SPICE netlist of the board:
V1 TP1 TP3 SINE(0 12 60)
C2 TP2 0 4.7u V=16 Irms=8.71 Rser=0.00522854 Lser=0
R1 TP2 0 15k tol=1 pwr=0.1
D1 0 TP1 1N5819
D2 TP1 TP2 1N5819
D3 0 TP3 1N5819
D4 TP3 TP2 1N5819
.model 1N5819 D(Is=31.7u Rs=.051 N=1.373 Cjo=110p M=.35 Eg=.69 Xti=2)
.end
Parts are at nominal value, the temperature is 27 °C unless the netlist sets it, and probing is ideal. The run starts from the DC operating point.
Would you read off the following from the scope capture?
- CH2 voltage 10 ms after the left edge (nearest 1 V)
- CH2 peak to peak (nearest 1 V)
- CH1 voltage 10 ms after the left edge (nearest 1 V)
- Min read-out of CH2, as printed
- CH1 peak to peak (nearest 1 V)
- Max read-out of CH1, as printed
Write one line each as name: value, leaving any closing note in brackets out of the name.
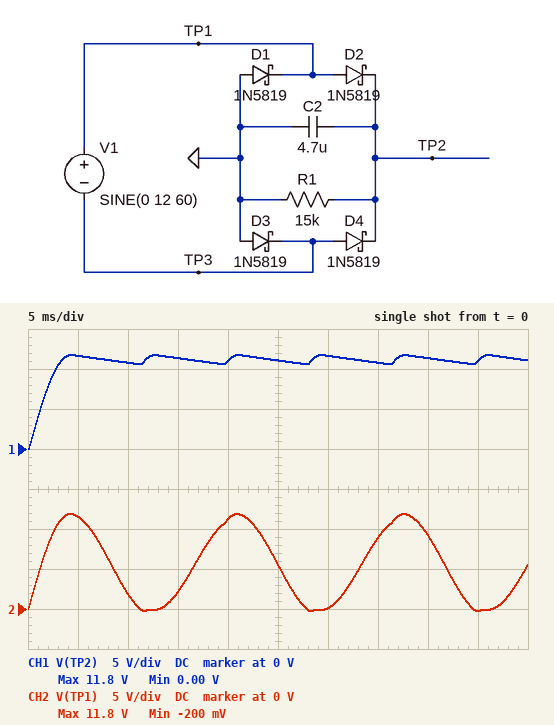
CH2 voltage 10 ms after the left edge: 2 V
CH2 peak to peak: 12 V
CH1 voltage 10 ms after the left edge: 11 V
Min read-out of CH2, as printed: -200 mV
CH1 peak to peak: 12 V
Max read-out of CH1, as printed: 11.8 V
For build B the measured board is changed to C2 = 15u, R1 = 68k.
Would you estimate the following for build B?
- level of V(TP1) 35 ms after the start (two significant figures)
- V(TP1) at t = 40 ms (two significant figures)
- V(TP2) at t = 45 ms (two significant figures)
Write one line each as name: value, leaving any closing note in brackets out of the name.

level of V(TP1) 35 ms after the start: 9.3 V
V(TP1) at t = 40 ms: 9.4 V
V(TP2) at t = 45 ms: 12 V
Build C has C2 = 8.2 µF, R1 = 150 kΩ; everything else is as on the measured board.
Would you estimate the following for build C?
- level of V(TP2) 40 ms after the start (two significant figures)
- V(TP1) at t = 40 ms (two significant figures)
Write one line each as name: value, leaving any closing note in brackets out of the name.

level of V(TP2) 40 ms after the start: 12 V
V(TP1) at t = 40 ms: 9.4 V
